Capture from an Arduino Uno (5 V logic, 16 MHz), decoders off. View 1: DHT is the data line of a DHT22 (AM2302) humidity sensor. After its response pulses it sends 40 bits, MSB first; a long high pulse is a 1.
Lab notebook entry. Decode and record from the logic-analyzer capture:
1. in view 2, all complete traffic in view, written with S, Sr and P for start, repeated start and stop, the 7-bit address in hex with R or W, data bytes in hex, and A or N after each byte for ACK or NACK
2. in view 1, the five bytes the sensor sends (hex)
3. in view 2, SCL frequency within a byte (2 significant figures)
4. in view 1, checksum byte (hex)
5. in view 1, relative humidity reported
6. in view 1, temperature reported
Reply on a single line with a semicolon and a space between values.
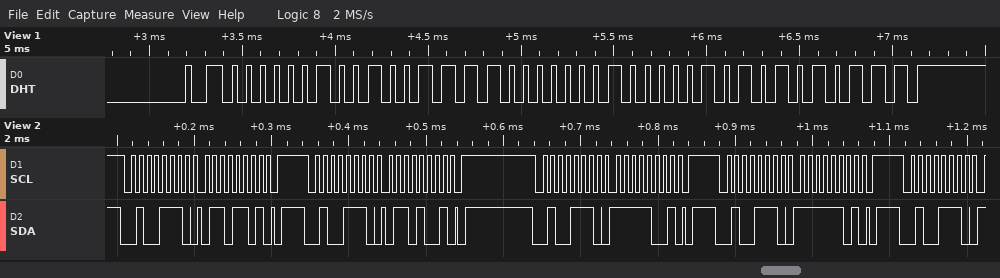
S 27W A 6D A P S 27W A 69 A P S 27W A F9 A P S 27W A FD A P S 27W A; 02 4F 01 05 57; 100 kHz; 0x57; 59.1 %; 26.1 °C
